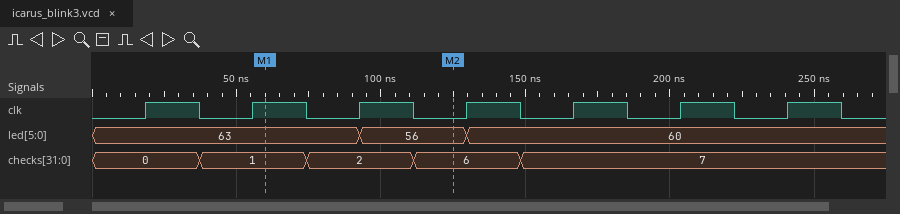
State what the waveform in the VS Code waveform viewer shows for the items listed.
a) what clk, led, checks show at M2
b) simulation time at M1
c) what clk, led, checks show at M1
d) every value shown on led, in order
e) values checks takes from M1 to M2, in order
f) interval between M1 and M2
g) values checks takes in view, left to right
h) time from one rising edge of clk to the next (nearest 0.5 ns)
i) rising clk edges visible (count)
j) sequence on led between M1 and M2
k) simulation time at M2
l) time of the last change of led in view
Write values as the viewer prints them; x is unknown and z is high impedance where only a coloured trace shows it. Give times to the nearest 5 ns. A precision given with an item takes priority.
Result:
clk=0, led=56, checks=6
60 ns
clk=1, led=63, checks=1
63, 56, 60
1, 2, 6
65 ns
0, 1, 2, 6, 7
37 ns
7
63, 56
125 ns
130 ns
